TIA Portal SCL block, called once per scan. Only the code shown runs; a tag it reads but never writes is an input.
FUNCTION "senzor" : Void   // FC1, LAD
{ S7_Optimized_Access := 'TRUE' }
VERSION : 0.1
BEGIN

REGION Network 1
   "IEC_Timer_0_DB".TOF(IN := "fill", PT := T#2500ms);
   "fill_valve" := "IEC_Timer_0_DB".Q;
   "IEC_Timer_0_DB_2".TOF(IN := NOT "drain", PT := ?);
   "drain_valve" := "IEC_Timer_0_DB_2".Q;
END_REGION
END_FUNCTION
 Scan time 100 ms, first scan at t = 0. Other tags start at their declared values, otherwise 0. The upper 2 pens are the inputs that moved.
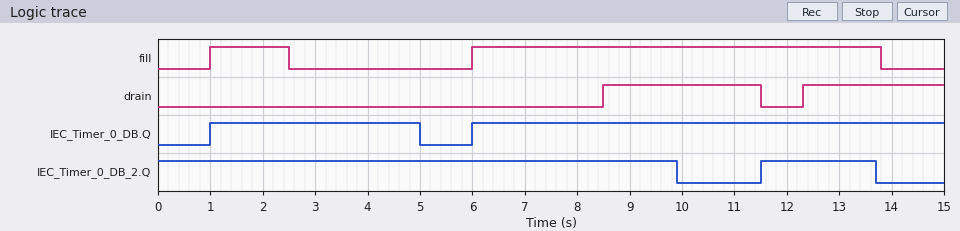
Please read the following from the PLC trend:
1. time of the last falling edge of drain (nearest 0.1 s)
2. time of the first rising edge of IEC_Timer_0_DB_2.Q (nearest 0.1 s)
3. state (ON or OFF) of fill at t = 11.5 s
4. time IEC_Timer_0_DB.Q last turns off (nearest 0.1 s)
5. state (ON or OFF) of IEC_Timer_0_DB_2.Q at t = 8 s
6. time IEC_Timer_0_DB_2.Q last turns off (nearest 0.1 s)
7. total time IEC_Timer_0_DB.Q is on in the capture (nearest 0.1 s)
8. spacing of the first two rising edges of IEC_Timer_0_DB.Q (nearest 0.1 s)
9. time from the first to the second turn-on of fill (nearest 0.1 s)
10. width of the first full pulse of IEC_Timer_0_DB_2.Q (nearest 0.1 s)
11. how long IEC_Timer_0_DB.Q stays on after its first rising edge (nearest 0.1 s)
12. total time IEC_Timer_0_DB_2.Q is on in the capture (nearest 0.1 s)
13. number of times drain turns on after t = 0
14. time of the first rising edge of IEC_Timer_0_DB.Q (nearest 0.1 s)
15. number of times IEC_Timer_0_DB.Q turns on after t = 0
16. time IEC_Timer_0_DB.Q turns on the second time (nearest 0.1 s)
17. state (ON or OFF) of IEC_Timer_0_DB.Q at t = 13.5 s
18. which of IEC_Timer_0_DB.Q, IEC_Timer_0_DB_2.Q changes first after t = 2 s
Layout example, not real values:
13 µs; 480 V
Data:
11.5 s; 11.5 s; ON; 5.0 s; ON; 13.7 s; 13.0 s; 5.0 s; 5.0 s; 2.2 s; 4.0 s; 12.1 s; 2; 1.0 s; 2; 6.0 s; ON; IEC_Timer_0_DB.Q
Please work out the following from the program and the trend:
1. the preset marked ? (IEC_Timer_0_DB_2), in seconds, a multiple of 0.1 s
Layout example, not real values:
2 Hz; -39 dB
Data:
1.4 s
